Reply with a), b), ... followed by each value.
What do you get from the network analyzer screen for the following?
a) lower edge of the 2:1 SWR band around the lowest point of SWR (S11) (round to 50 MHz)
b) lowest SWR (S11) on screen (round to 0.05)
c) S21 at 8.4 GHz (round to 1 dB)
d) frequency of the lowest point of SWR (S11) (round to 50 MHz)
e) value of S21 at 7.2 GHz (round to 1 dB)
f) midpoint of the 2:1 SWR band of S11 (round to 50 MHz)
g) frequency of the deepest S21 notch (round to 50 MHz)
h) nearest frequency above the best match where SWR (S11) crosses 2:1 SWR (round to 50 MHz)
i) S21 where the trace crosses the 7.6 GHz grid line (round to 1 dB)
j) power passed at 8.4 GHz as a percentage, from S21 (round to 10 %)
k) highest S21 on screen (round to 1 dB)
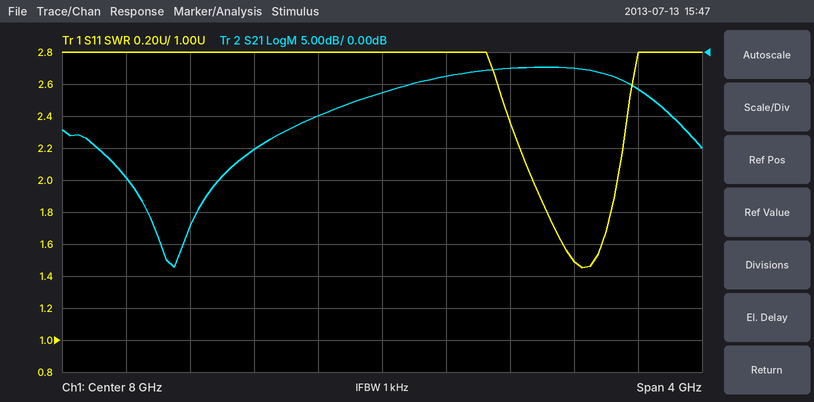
a) 8.95 GHz
b) 1.45
c) -4 dB
d) 9.25 GHz
e) -15 dB
f) 9.20 GHz
g) 6.70 GHz
h) 9.45 GHz
i) -10 dB
j) 40 %
k) -2 dB
